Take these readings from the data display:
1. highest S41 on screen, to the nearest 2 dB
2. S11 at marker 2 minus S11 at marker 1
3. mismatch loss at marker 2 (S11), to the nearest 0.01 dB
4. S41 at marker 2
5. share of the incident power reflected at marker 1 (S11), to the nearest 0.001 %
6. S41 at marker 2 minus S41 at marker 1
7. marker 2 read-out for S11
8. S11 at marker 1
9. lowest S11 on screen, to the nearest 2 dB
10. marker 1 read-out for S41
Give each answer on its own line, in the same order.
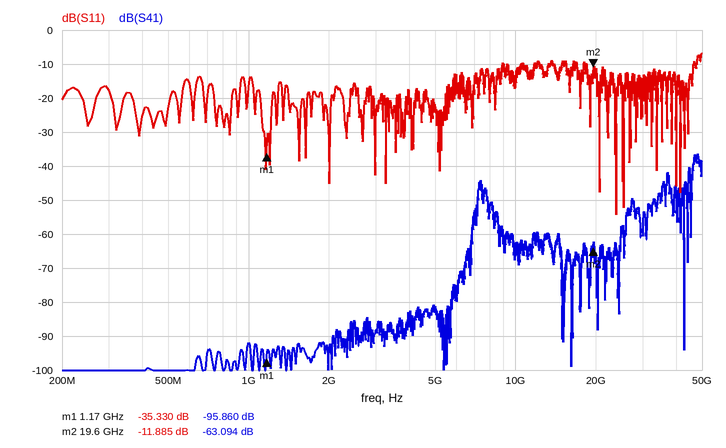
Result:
-36 dB
23.445 dB
0.29 dB
-63.094 dB
0.029 %
32.766 dB
-11.885 dB
-35.330 dB
-54 dB
-95.860 dB
